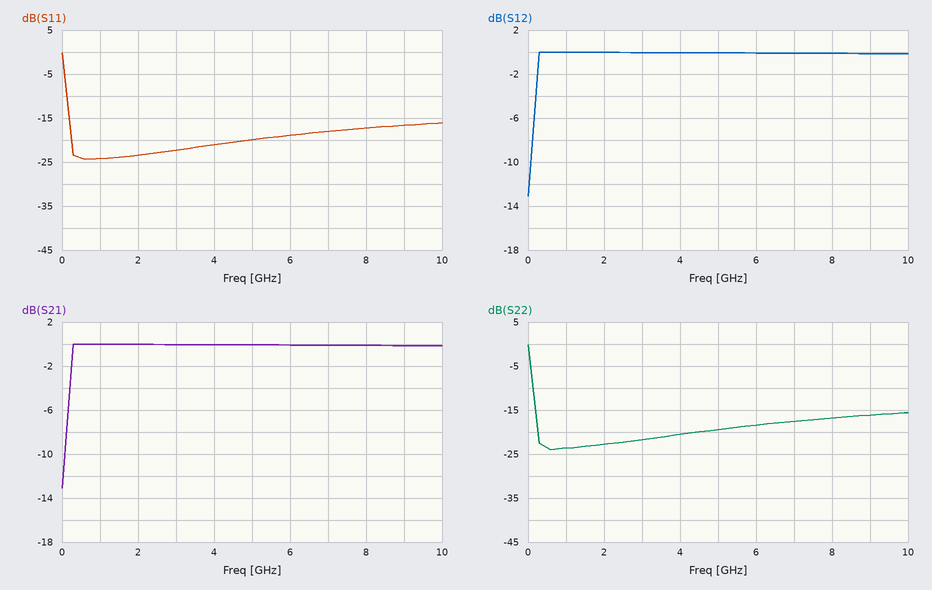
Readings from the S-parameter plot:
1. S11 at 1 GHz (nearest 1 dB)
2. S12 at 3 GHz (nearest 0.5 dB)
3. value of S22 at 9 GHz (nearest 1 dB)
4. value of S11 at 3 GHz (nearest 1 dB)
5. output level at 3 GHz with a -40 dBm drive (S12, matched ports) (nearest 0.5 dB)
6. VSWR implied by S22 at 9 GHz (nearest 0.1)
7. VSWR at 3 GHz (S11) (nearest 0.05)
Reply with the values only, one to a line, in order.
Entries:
-24 dB
0.0 dB
-16 dB
-22 dB
-40.0 dBm
1.4
1.15
